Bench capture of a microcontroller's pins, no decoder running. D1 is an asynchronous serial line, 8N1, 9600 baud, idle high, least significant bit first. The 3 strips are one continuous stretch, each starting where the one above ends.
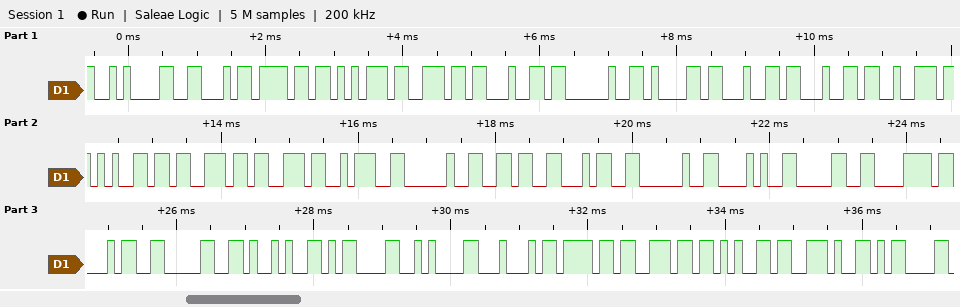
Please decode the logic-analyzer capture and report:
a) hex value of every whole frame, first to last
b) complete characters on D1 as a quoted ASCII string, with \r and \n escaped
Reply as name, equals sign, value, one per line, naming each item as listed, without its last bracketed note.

hex value of every whole frame, first to last = 0A 46 6F 75 6E 64 20 61 64 64 72 65 73 73 3A 20 36 34 20 28 30 78 34 30 29 0D 0A 44 6F 6E 65 2E 0D
complete characters on D1 as a quoted ASCII string, with \r and \n escaped = "\nFound address: 64 (0x40)\r\nDone.\r"
